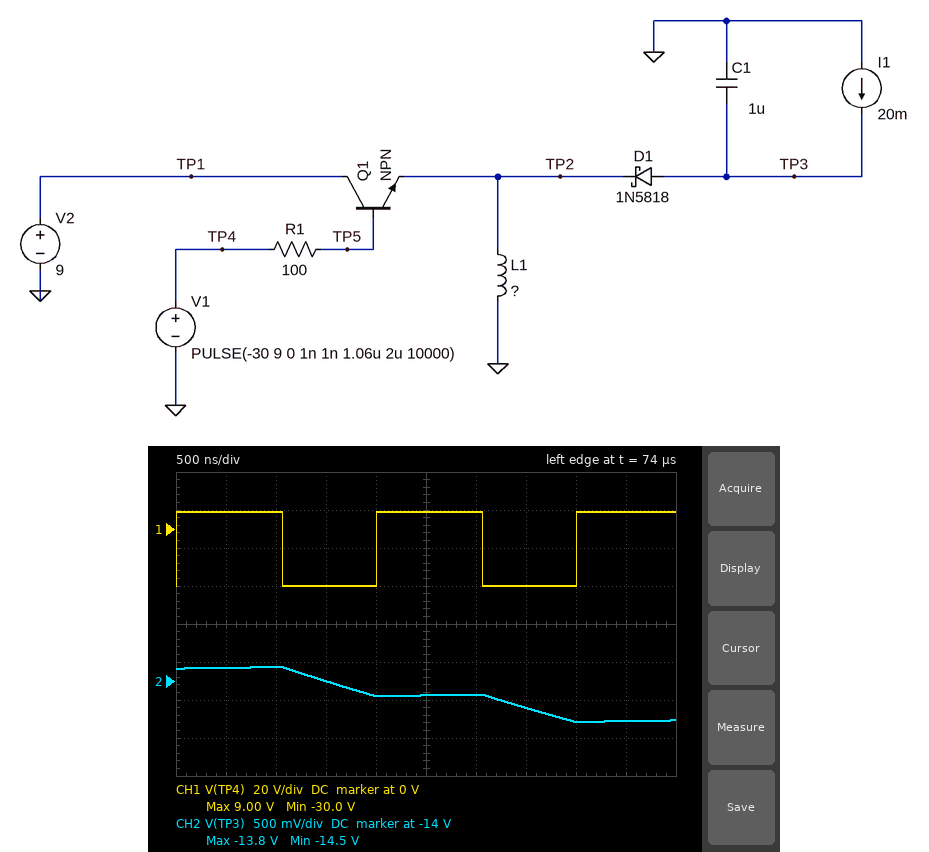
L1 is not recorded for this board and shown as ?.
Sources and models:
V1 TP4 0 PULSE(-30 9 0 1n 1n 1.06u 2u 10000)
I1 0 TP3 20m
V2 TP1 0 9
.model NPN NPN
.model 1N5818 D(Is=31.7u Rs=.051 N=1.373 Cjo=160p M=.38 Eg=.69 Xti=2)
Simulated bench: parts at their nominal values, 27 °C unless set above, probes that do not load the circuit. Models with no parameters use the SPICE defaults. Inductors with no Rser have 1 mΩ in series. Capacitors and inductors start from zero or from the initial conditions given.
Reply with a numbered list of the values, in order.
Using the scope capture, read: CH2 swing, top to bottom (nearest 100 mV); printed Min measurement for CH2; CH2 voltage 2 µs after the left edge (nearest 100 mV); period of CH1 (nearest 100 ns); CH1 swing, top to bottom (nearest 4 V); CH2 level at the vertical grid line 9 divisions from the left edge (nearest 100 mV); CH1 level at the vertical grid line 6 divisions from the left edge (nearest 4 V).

1. 700 mV
2. -14.5 V
3. -14.2 V
4. 2.0 µs
5. 40 V
6. -14.5 V
7. 8 V
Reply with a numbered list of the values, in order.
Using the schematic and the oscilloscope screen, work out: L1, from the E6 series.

1. 220 µH
